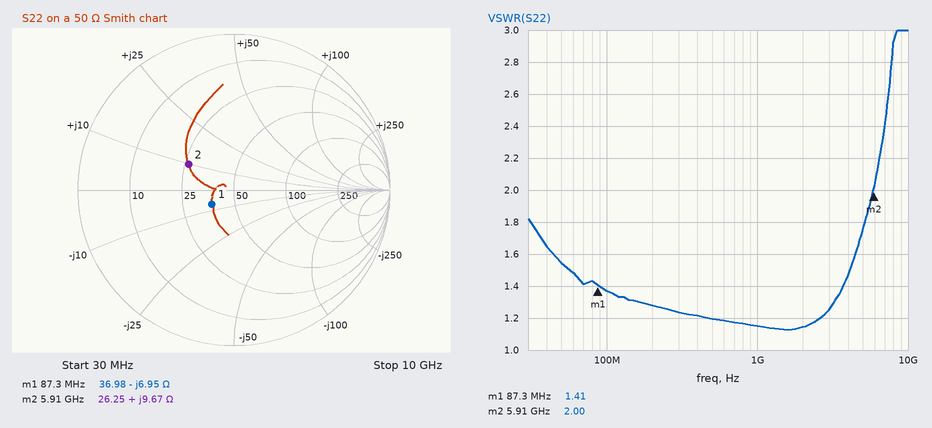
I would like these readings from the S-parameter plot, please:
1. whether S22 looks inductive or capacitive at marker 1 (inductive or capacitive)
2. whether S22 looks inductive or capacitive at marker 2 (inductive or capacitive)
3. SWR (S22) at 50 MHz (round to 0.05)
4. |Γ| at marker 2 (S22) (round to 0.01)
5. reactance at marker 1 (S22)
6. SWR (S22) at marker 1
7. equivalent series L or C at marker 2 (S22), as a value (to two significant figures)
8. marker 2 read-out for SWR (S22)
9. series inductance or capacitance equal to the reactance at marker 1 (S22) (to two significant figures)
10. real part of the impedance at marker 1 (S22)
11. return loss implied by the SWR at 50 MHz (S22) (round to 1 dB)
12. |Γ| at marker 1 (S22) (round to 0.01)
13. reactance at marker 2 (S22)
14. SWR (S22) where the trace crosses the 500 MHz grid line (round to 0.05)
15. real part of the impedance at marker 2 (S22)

capacitive
inductive
1.55
0.33
-6.95 Ω
1.41
260 pH
2.00
260 pF
36.98 Ω
13 dB
0.17
+9.67 Ω
1.20
26.25 Ω
